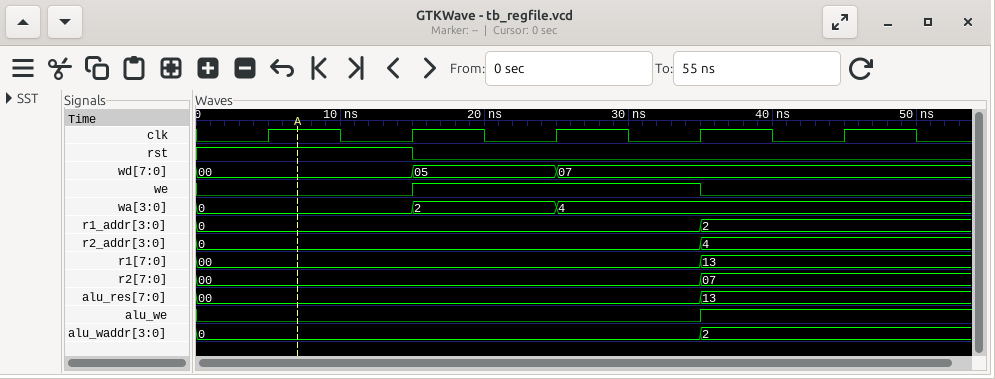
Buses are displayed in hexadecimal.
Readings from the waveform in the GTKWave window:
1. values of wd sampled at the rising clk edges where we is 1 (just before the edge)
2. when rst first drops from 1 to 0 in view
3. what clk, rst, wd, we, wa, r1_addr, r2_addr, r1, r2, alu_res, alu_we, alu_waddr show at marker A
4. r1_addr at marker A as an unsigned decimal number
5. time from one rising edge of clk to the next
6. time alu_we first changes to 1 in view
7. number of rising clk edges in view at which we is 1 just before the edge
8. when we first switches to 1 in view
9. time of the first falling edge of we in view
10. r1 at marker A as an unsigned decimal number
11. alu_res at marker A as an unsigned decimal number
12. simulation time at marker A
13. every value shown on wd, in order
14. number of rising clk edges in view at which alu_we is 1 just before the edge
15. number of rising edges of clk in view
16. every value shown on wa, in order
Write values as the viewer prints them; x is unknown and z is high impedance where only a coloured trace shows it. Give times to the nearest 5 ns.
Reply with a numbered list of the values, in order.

1. 05, 07
2. 15 ns
3. clk=1, rst=1, wd=00, we=0, wa=0, r1_addr=0, r2_addr=0, r1=00, r2=00, alu_res=00, alu_we=0, alu_waddr=0
4. 0
5. 10 ns
6. 35 ns
7. 2
8. 15 ns
9. 35 ns
10. 0
11. 0
12. 5 ns
13. 00, 05, 07
14. 1
15. 5
16. 0, 2, 4
